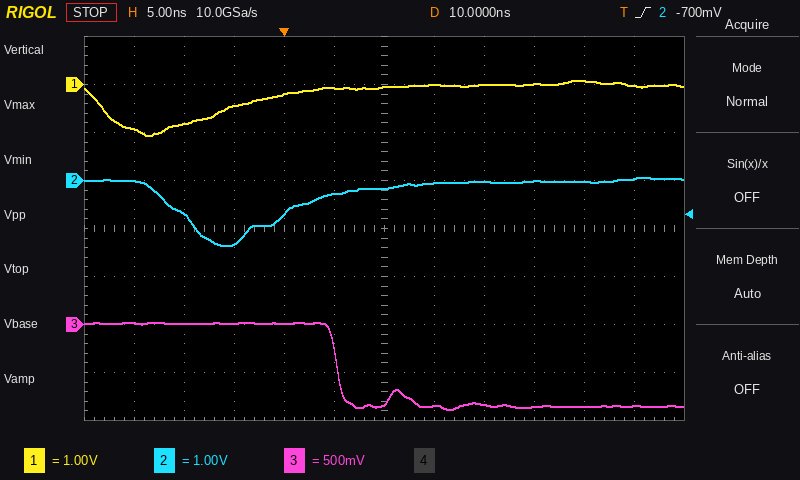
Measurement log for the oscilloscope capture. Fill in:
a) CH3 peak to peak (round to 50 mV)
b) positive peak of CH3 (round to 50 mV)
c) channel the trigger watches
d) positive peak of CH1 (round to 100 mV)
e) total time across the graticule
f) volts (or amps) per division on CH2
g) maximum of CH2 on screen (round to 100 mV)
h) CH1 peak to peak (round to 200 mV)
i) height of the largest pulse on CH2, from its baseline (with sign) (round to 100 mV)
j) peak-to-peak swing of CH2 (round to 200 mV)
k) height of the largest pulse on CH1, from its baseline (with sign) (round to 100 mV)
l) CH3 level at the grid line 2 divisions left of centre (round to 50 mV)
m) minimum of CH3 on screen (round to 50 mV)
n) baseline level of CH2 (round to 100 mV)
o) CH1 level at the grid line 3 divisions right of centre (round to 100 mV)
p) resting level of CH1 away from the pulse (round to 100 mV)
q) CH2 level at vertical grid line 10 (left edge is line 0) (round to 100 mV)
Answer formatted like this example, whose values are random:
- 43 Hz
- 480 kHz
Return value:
- 900 mV
- 0 mV
- CH2
- 100 mV
- 60 ns
- 1 V
- 100 mV
- 1.2 V
- -1.3 V
- 1.4 V
- -1.0 V
- 0 mV
- -900 mV
- 0.0 V
- 0.0 V
- 0.0 V
- 0.0 V
